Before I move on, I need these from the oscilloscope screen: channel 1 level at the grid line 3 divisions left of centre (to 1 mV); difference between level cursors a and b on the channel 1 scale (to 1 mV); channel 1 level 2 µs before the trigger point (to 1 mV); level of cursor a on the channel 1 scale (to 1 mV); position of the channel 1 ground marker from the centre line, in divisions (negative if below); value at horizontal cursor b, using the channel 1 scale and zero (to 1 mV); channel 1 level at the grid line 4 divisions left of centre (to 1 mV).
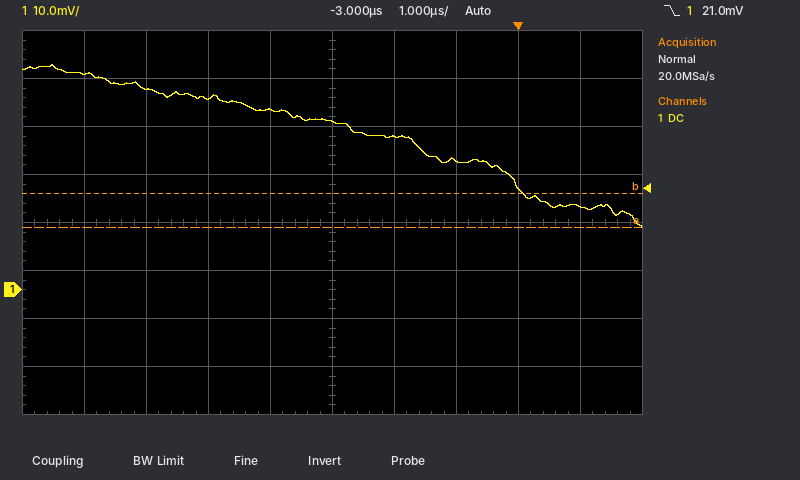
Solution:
42 mV
7 mV
32 mV
13 mV
-1.4 div
20 mV
45 mV
